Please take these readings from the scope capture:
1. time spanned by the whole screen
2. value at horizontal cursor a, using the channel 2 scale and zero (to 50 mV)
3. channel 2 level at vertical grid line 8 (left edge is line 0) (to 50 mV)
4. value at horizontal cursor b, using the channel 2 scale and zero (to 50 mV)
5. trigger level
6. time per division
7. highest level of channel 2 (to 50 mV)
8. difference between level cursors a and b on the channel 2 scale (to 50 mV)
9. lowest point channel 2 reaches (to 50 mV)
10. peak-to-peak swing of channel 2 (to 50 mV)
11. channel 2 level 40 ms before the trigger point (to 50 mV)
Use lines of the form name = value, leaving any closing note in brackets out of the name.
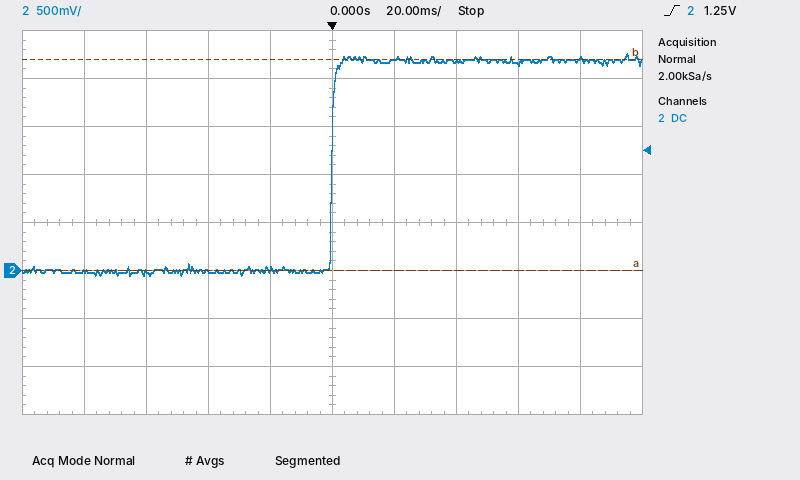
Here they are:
time spanned by the whole screen = 200 ms
value at horizontal cursor a, using the channel 2 scale and zero = 0 mV
channel 2 level at vertical grid line 8 (left edge is line 0) = 2.15 V
value at horizontal cursor b, using the channel 2 scale and zero = 2.20 V
trigger level = 1.25 V
time per division = 20 ms
highest level of channel 2 = 2.25 V
difference between level cursors a and b on the channel 2 scale = 2.20 V
lowest point channel 2 reaches = -50 mV
peak-to-peak swing of channel 2 = 2.30 V
channel 2 level 40 ms before the trigger point = 0 mV
